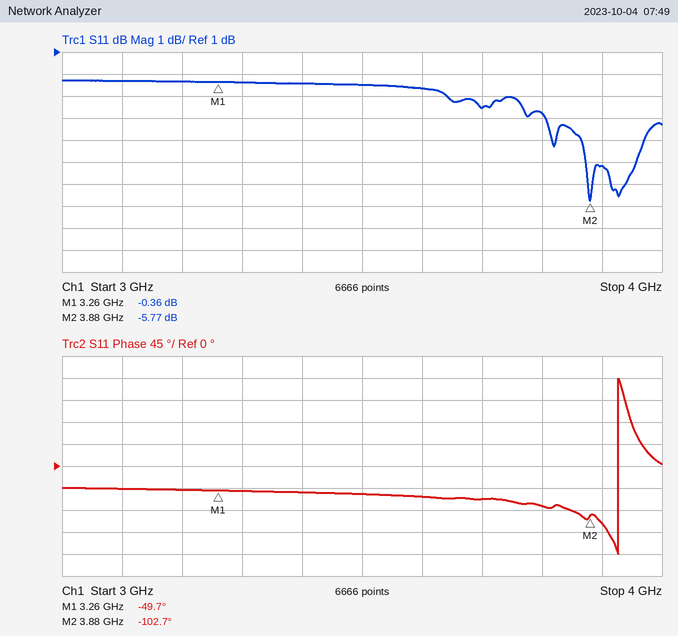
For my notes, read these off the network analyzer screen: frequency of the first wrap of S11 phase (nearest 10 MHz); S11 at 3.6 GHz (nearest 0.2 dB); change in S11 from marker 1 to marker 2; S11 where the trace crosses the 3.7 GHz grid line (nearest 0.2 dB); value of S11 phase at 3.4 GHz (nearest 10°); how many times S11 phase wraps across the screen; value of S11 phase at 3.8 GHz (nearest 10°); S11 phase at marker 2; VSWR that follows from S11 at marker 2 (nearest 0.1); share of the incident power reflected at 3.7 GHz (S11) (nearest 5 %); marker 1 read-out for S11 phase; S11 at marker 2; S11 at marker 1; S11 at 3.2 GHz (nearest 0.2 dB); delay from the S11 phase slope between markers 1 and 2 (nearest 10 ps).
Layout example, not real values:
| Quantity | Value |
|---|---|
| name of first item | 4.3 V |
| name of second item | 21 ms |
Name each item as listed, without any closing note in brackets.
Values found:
| Quantity | Value |
|---|---|
| frequency of the first wrap of S11 phase | 3.93 GHz |
| S11 at 3.6 GHz | -0.6 dB |
| change in S11 from marker 1 to marker 2 | -5.41 dB |
| S11 where the trace crosses the 3.7 GHz grid line | -1.6 dB |
| value of S11 phase at 3.4 GHz | -50° |
| how many times S11 phase wraps across the screen | 1 |
| value of S11 phase at 3.8 GHz | -80° |
| S11 phase at marker 2 | -102.7° |
| VSWR that follows from S11 at marker 2 | 3.1 |
| share of the incident power reflected at 3.7 GHz (S11) | 70 % |
| marker 1 read-out for S11 phase | -49.7° |
| S11 at marker 2 | -5.77 dB |
| S11 at marker 1 | -0.36 dB |
| S11 at 3.2 GHz | -0.4 dB |
| delay from the S11 phase slope between markers 1 and 2 | 240 ps |
